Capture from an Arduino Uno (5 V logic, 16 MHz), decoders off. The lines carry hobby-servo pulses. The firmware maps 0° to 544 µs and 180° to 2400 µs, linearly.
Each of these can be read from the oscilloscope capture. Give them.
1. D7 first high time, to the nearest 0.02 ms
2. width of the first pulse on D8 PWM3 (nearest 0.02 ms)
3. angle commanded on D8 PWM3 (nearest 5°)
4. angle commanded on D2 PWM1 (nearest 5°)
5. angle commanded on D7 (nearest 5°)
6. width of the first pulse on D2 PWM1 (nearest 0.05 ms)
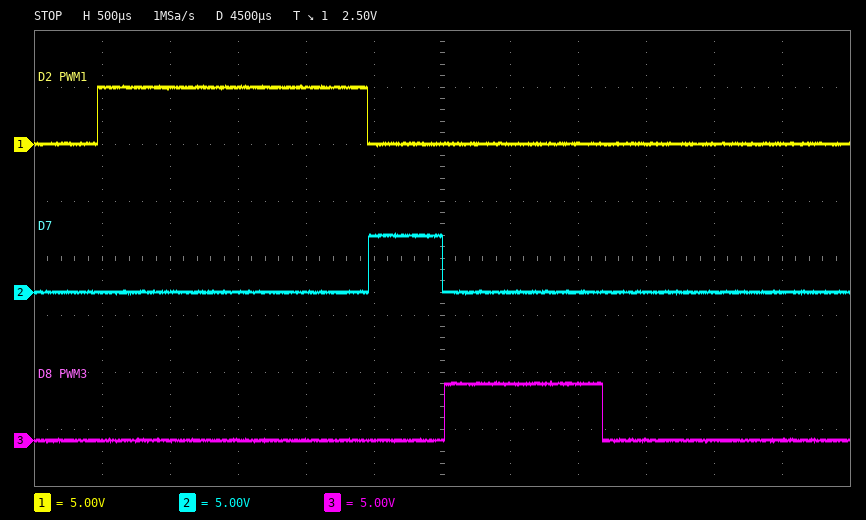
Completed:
0.54 ms
1.16 ms
60°
140°
0°
2.00 ms
